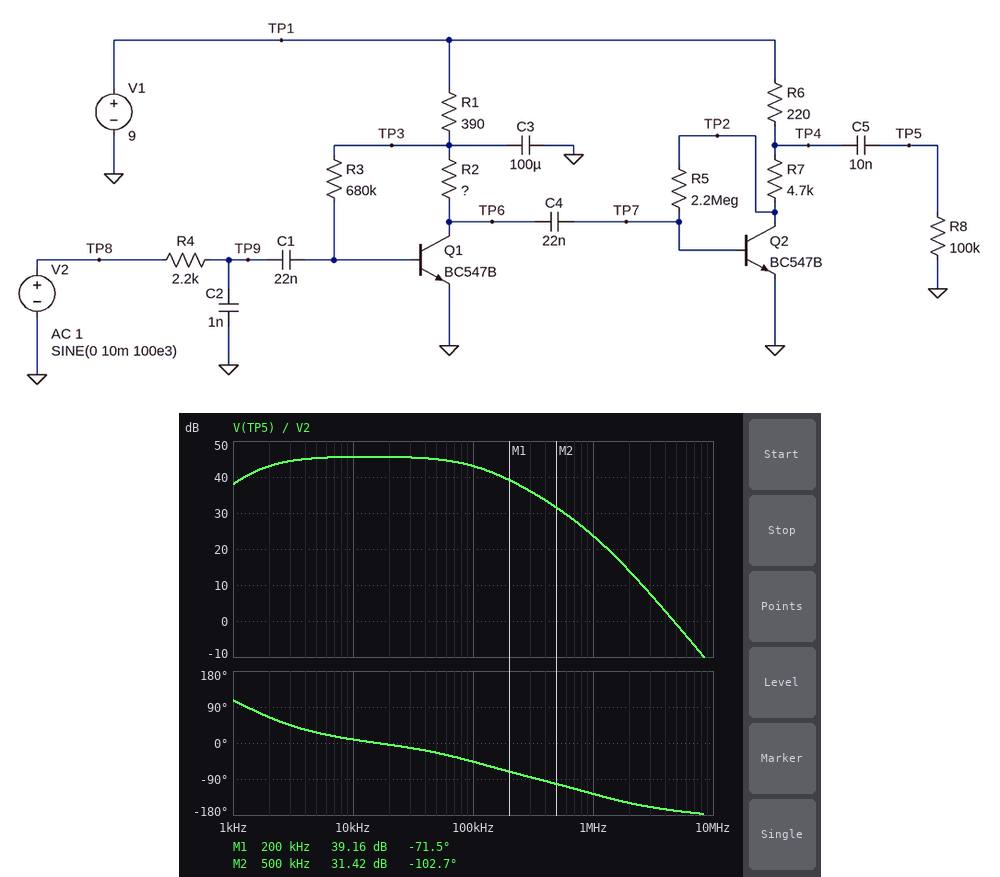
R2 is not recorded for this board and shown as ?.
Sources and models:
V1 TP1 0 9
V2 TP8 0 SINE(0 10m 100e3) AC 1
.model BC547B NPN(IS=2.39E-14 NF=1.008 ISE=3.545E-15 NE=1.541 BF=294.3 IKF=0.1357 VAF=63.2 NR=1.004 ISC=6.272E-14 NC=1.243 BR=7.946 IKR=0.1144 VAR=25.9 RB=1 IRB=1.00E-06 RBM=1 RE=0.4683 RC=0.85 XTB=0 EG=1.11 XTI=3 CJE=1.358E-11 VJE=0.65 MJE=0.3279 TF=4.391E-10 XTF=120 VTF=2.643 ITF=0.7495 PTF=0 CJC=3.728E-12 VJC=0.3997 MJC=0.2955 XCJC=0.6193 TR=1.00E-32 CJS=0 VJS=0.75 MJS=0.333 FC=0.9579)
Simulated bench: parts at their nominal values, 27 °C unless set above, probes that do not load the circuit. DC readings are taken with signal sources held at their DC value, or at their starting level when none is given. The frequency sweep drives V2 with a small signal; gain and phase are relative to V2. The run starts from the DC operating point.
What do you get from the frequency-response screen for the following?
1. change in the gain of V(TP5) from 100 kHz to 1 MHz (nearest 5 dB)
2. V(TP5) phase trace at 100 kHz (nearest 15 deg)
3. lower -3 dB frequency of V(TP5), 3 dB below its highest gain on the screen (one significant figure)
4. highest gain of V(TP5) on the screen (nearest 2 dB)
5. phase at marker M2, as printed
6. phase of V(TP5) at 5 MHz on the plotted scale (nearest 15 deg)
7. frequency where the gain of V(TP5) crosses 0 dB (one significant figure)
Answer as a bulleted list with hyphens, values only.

- -20 dB
- -45 deg
- 2 kHz
- 46 dB
- -102.7 deg
- -165 deg
- 5 MHz
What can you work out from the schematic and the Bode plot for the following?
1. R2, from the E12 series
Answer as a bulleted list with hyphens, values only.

- 680 Ω
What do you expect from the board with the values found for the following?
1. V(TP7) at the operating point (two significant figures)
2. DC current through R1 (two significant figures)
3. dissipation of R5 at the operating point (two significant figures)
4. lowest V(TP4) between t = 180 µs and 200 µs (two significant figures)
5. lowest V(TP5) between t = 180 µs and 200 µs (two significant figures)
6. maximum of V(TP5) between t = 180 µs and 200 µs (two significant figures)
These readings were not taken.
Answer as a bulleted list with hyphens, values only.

- 630 mV
- 3.2 mA
- 11 µW
- 8.6 V
- -250 mV
- 150 mV
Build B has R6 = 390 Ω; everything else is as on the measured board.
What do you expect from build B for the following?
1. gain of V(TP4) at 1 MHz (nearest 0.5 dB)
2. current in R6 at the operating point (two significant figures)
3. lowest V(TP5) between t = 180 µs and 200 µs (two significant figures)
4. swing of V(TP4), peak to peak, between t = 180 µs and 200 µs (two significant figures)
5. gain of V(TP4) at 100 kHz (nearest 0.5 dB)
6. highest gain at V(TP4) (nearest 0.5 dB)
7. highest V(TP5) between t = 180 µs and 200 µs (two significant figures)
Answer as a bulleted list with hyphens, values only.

- 28.5 dB
- 680 µA
- -430 mV
- 680 mV
- 48.0 dB
- 50.5 dB
- 260 mV
